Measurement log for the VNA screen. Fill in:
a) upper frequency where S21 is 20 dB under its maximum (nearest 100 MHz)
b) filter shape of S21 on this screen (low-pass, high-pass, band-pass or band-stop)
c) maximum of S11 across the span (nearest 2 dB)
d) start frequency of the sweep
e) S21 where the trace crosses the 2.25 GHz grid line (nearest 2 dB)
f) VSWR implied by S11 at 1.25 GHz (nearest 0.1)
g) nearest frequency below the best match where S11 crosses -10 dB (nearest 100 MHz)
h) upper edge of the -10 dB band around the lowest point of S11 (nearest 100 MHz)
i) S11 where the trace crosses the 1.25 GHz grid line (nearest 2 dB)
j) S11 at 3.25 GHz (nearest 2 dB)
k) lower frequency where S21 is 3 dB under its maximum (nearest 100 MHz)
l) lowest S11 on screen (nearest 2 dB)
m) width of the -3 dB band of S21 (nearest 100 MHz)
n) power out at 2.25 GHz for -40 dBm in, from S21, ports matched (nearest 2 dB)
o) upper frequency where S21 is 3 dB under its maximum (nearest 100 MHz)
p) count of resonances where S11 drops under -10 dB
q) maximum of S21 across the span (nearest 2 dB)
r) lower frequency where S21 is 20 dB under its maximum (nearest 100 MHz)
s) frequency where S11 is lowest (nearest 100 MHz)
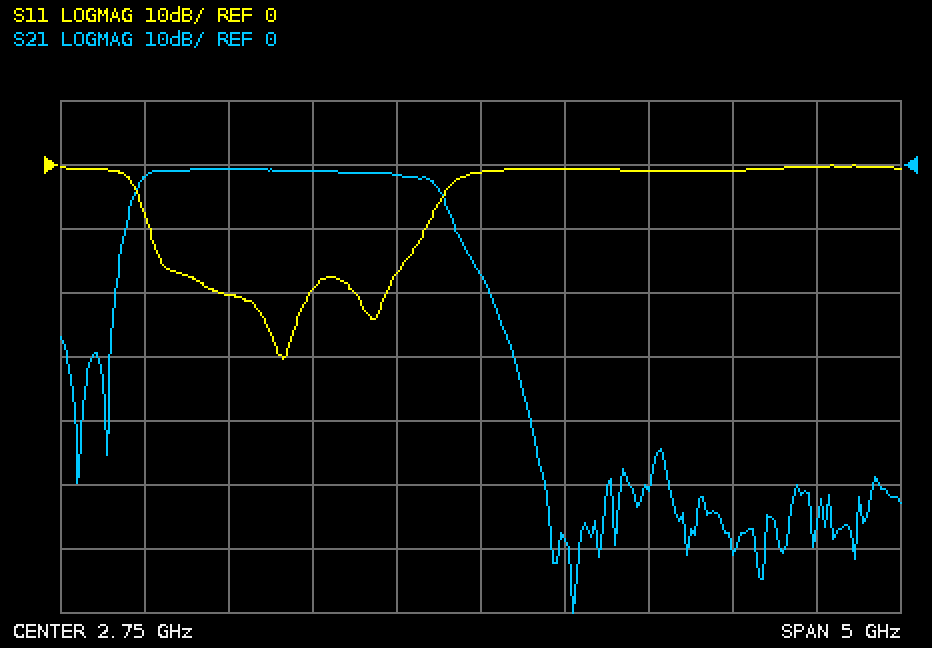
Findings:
2.8 GHz
band-pass
0 dB
250 MHz
-2 dB
1.2
800 MHz
2.4 GHz
-20 dB
0 dB
700 MHz
-30 dB
1.8 GHz
-42 dBm
2.5 GHz
2
0 dB
600 MHz
1.6 GHz
